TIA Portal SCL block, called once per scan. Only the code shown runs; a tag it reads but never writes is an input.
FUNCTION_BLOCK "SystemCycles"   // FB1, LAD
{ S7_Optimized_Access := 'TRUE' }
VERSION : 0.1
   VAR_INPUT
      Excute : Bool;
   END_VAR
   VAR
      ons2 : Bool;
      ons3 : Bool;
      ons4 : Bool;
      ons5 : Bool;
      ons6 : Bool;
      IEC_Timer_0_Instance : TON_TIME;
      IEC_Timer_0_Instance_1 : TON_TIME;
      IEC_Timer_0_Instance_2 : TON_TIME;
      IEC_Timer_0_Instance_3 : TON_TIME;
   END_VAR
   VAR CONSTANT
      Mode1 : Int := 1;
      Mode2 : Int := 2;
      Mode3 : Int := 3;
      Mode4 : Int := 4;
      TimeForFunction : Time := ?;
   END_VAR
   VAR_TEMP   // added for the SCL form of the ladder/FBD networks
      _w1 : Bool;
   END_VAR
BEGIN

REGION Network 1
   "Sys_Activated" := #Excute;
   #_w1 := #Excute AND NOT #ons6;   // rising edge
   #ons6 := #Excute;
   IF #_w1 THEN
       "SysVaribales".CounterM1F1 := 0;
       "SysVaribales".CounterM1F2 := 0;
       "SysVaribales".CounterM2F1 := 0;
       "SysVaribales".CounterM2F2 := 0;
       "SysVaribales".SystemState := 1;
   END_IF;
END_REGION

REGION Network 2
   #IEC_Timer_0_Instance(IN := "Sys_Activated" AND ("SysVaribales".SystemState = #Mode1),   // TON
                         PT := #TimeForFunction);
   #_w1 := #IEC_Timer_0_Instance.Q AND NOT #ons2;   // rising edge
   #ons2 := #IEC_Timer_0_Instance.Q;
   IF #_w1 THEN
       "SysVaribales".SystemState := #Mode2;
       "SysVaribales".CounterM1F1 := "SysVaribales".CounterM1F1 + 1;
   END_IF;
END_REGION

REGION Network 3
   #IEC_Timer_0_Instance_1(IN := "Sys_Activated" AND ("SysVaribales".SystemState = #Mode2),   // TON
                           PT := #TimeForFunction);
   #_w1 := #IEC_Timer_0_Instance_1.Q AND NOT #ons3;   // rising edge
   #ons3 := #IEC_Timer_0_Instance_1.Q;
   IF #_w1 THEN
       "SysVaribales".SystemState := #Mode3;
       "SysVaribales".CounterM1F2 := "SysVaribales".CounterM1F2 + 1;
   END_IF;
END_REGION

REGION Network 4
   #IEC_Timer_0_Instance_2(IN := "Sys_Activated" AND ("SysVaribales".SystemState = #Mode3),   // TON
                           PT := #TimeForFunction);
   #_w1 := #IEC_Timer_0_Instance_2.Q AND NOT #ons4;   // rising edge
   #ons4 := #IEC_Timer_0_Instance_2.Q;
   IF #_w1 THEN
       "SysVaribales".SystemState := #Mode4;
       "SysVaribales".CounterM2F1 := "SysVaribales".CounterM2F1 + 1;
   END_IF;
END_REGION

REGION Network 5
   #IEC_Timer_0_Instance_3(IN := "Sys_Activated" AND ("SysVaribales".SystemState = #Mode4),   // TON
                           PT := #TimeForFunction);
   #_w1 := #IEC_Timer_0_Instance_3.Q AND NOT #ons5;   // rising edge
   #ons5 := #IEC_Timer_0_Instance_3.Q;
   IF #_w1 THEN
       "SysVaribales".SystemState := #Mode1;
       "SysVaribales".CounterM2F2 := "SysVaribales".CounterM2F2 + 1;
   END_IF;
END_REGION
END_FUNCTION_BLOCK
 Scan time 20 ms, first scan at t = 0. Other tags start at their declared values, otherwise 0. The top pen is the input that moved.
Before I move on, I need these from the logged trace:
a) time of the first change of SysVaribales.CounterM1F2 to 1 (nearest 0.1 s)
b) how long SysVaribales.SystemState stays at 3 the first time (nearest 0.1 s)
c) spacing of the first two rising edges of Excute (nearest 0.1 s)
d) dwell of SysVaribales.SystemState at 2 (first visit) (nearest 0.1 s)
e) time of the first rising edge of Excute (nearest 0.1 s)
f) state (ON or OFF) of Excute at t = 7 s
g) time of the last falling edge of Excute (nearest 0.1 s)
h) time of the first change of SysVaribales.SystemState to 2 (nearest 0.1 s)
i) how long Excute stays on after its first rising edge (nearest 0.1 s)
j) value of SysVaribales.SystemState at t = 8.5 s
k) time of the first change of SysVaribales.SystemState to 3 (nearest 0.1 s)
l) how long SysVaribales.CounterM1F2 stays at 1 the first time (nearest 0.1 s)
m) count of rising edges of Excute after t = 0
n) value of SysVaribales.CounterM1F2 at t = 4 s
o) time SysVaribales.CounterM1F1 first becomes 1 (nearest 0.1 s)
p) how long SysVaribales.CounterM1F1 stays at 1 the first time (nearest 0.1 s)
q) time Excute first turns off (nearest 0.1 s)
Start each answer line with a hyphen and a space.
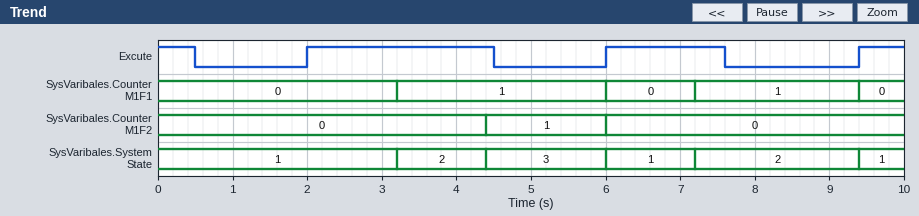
- 4.4 s
- 1.6 s
- 4.0 s
- 1.2 s
- 2.0 s
- ON
- 7.6 s
- 3.2 s
- 2.5 s
- 2
- 4.4 s
- 1.6 s
- 3
- 0
- 3.2 s
- 2.8 s
- 0.5 s
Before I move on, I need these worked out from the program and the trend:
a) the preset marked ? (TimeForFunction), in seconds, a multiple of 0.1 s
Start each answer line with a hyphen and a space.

- 1.2 s
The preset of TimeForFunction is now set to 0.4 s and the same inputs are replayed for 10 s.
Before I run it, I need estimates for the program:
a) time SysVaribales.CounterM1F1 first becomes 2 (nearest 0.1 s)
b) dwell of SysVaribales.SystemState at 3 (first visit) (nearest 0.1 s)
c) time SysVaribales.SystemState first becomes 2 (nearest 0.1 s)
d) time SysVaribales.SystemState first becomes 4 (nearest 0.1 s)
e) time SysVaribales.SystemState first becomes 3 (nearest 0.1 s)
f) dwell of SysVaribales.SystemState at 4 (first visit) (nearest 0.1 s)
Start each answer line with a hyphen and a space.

- 4.0 s
- 0.4 s
- 0.4 s
- 3.2 s
- 2.8 s
- 0.4 s
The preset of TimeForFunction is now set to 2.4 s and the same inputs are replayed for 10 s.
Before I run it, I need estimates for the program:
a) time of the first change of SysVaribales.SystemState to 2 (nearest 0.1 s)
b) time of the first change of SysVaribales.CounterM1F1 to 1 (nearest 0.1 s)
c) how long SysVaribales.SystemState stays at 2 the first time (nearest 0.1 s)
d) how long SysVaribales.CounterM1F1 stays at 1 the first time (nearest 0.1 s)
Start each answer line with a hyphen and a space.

- 4.4 s
- 4.4 s
- 1.6 s
- 1.6 s
